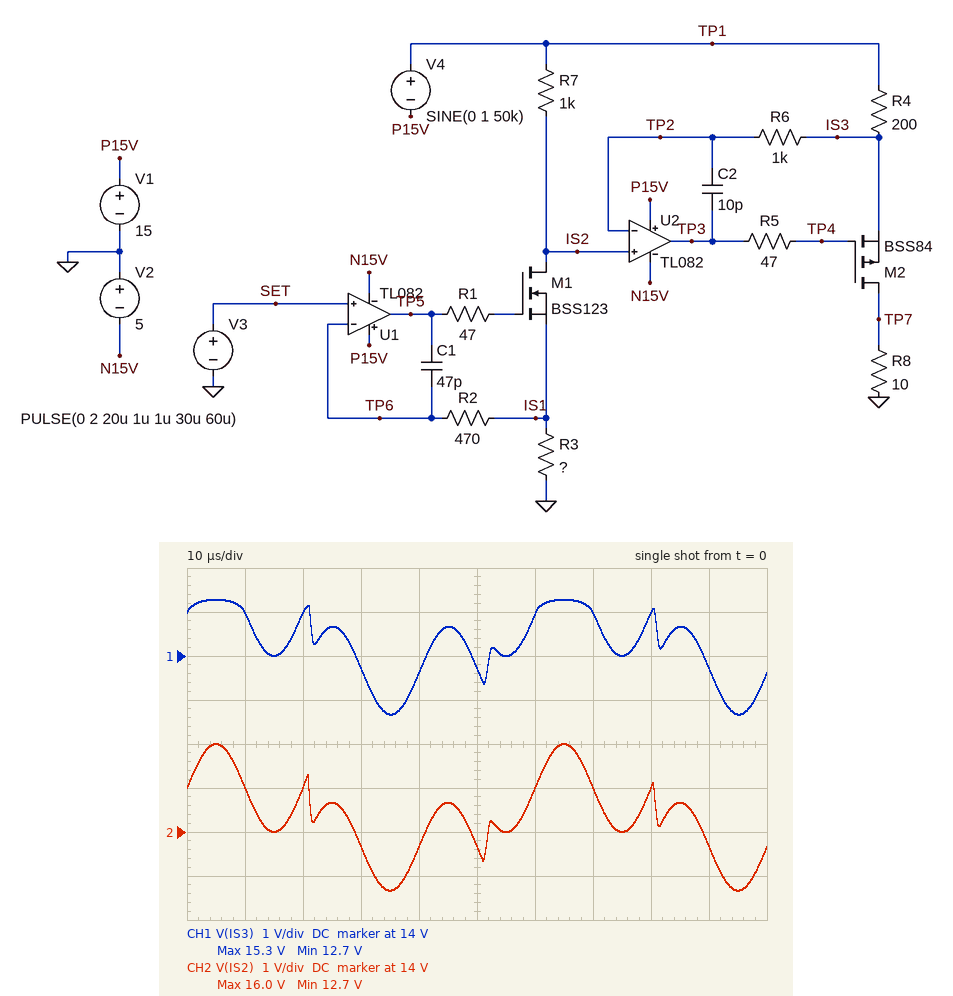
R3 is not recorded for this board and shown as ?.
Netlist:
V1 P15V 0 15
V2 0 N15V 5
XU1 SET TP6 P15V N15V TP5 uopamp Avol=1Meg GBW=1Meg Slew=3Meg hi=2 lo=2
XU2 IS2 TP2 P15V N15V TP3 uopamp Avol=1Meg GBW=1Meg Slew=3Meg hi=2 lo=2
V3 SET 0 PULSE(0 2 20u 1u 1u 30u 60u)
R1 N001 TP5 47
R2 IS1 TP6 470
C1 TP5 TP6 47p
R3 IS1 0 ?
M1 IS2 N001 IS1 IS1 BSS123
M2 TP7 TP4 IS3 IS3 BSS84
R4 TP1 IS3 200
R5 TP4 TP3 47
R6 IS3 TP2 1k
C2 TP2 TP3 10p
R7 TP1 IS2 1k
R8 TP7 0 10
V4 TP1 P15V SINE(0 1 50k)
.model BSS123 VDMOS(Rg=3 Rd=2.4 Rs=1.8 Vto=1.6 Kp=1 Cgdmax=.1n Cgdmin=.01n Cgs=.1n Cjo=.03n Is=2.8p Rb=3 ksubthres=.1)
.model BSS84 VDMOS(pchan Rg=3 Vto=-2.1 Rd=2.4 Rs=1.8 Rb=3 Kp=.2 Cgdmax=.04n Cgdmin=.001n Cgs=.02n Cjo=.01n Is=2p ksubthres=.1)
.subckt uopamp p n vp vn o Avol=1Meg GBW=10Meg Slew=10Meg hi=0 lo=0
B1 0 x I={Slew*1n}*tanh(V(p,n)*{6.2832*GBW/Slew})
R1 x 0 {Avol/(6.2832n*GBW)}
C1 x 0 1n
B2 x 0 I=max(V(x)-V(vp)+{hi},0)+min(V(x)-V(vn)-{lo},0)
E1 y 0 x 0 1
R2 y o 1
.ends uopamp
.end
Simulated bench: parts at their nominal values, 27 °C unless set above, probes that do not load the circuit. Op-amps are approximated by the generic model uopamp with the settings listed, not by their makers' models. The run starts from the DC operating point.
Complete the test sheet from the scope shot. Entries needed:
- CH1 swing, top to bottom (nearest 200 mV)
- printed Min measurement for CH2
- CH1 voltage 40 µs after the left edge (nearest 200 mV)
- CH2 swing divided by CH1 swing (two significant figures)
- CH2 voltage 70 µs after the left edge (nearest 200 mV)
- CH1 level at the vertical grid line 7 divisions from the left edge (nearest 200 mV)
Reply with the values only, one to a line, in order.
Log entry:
2.6 V
12.7 V
13.6 V
1.3
15.0 V
15.0 V
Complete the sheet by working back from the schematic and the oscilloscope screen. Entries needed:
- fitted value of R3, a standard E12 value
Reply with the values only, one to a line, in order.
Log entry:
1.5 kΩ
